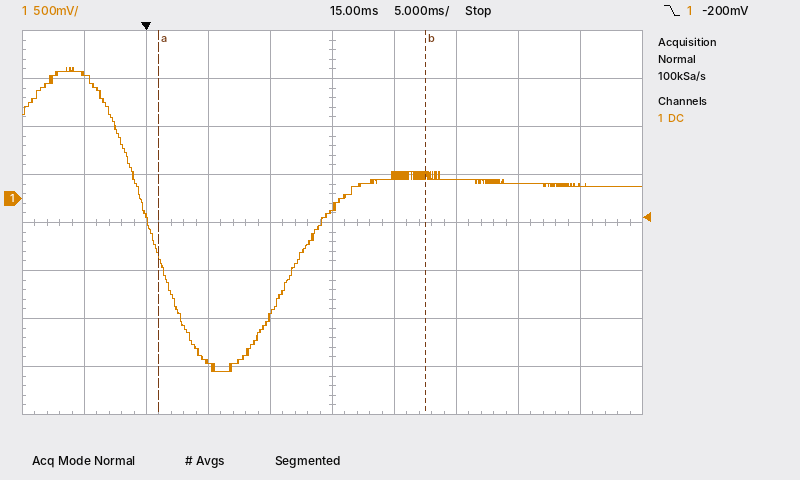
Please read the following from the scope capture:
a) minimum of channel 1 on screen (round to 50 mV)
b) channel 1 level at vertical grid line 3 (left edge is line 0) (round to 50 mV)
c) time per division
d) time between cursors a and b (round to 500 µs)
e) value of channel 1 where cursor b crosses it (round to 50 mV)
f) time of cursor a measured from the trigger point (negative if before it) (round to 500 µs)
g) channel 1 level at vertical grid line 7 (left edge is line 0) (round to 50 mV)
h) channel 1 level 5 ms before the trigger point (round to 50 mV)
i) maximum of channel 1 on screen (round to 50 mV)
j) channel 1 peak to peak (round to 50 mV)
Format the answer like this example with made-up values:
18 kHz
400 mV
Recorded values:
-1.80 V
-1.70 V
5 ms
21.5 ms
250 mV
+1.0 ms
200 mV
1.30 V
1.35 V
3.15 V
